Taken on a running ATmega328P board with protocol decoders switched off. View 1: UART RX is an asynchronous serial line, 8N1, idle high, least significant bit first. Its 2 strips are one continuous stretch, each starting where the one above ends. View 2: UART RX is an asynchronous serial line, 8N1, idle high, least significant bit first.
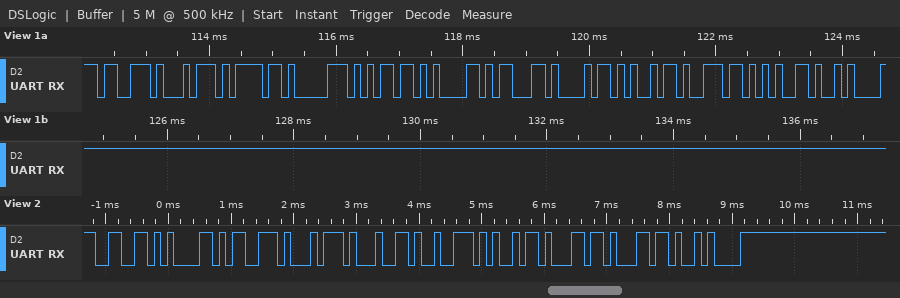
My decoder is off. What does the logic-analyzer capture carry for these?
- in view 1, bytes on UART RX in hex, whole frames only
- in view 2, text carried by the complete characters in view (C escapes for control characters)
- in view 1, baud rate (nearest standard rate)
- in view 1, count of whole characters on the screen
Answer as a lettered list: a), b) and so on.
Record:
a) 73 74 6F 70 6D 61 63 68 69 6E 65 0A
b) "fastdrill\n"
c) 9600 baud
d) 12
